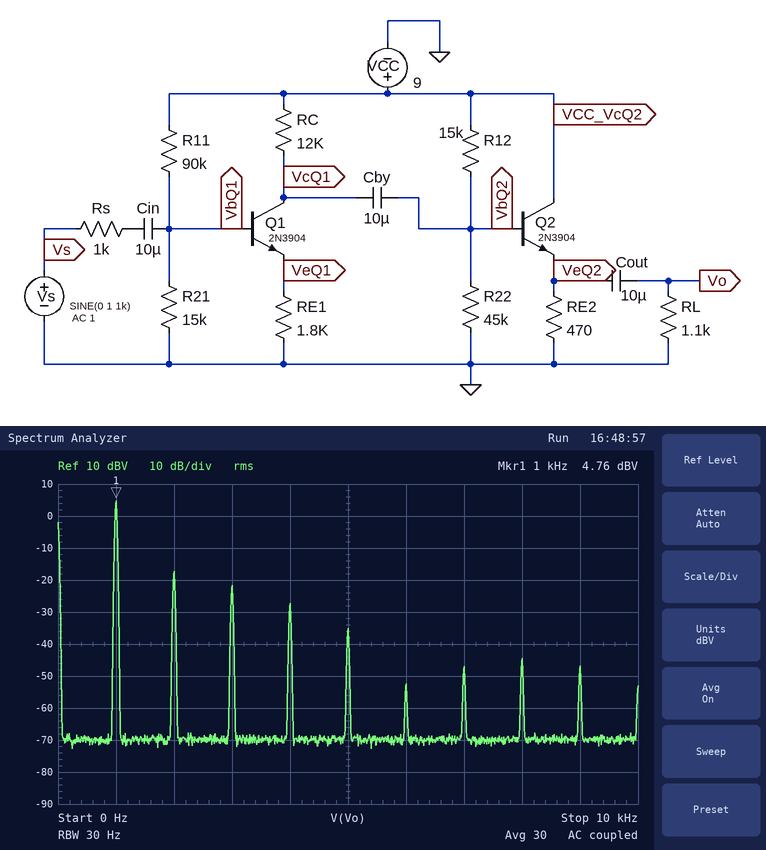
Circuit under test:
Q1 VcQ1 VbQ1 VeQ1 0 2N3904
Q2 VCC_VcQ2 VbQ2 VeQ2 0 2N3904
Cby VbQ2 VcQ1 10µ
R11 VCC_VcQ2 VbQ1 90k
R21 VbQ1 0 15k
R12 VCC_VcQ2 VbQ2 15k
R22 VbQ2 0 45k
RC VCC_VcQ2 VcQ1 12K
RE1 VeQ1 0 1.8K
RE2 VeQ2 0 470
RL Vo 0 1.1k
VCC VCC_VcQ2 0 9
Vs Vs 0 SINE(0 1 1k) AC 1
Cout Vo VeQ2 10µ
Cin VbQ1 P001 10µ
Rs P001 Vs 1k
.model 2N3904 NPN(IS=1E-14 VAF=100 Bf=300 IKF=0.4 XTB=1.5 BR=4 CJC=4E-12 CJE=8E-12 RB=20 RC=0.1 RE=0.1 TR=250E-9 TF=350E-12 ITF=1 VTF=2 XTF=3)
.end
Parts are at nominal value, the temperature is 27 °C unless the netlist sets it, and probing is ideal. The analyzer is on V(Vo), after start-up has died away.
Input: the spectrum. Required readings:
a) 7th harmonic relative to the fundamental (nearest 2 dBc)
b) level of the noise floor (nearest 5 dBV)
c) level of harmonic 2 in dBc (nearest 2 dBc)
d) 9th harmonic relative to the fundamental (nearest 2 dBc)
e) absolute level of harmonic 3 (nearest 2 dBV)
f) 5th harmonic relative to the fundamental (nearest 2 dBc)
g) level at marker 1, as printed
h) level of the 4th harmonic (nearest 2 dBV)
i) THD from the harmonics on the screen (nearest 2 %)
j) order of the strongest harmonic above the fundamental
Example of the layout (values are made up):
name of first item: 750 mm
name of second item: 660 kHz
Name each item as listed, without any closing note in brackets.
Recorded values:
7th harmonic relative to the fundamental: -52 dBc
level of the noise floor: -70 dBV
level of harmonic 2 in dBc: -22 dBc
9th harmonic relative to the fundamental: -52 dBc
absolute level of harmonic 3: -22 dBV
5th harmonic relative to the fundamental: -40 dBc
level at marker 1, as printed: 4.76 dBV
level of the 4th harmonic: -28 dBV
THD from the harmonics on the screen: 10 %
order of the strongest harmonic above the fundamental: 2
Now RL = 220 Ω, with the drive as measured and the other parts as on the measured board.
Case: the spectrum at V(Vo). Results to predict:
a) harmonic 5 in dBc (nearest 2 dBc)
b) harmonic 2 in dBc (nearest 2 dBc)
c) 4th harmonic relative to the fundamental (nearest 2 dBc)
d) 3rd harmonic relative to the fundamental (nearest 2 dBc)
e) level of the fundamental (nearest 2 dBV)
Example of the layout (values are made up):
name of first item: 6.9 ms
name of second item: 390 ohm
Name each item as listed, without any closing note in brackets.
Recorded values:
harmonic 5 in dBc: -32 dBc
harmonic 2 in dBc: -44 dBc
4th harmonic relative to the fundamental: -42 dBc
3rd harmonic relative to the fundamental: -18 dBc
level of the fundamental: 4 dBV
